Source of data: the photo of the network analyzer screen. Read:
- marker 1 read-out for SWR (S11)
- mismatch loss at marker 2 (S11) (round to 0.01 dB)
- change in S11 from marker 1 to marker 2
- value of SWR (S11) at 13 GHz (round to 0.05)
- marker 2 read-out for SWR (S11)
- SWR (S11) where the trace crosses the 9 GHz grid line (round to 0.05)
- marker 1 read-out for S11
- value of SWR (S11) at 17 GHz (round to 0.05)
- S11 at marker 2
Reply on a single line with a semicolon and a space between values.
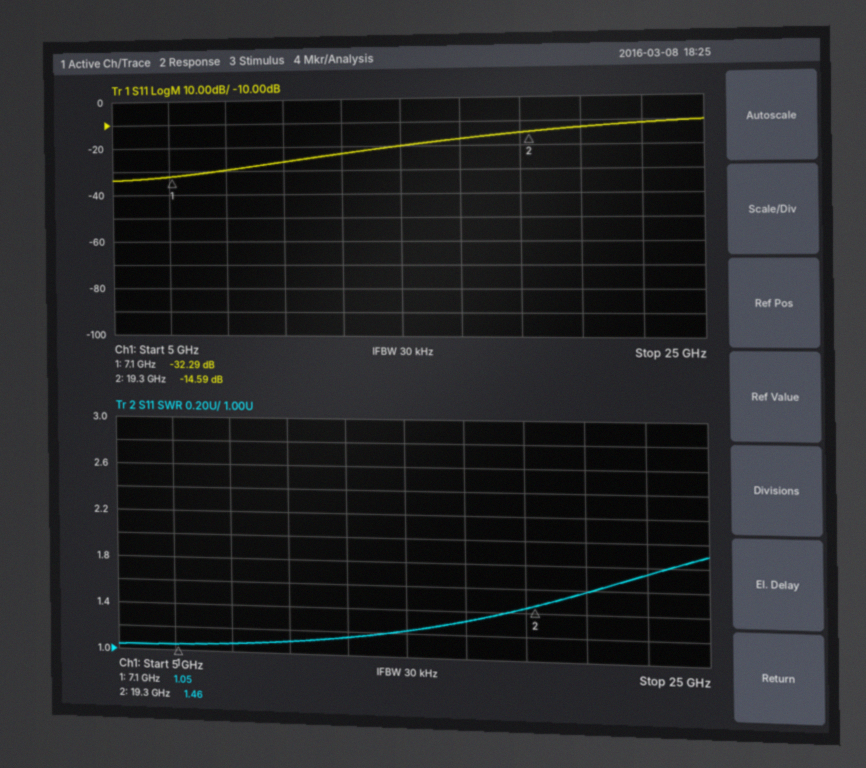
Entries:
1.05; 0.15 dB; 17.70 dB; 1.15; 1.46; 1.05; -32.29 dB; 1.30; -14.59 dB
